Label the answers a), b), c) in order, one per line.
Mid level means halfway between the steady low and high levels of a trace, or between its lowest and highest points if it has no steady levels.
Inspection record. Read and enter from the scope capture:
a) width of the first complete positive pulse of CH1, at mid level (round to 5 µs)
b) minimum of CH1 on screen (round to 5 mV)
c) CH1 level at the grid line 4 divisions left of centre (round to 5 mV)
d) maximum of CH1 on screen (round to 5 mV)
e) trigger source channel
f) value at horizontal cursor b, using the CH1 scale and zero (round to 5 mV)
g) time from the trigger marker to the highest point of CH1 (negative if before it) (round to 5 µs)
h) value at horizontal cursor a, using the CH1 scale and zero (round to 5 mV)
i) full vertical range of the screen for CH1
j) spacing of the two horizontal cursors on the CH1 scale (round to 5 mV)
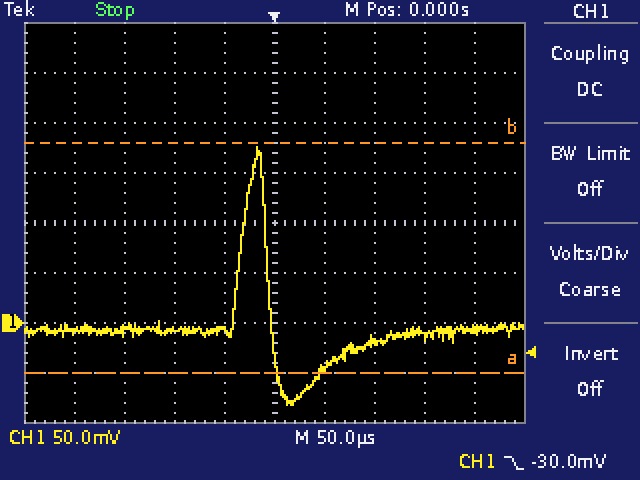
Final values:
a) 30 µs
b) -80 mV
c) -10 mV
d) 175 mV
e) CH1
f) 180 mV
g) -15 µs
h) -50 mV
i) 400 mV
j) 230 mV
